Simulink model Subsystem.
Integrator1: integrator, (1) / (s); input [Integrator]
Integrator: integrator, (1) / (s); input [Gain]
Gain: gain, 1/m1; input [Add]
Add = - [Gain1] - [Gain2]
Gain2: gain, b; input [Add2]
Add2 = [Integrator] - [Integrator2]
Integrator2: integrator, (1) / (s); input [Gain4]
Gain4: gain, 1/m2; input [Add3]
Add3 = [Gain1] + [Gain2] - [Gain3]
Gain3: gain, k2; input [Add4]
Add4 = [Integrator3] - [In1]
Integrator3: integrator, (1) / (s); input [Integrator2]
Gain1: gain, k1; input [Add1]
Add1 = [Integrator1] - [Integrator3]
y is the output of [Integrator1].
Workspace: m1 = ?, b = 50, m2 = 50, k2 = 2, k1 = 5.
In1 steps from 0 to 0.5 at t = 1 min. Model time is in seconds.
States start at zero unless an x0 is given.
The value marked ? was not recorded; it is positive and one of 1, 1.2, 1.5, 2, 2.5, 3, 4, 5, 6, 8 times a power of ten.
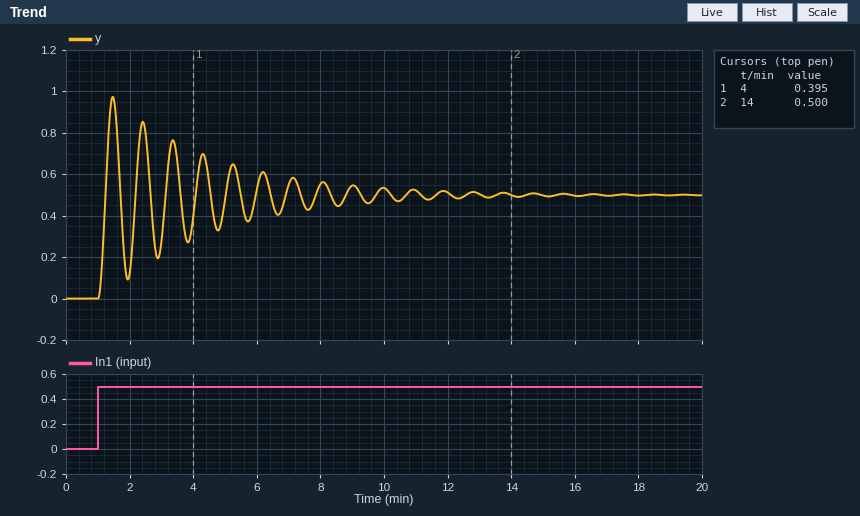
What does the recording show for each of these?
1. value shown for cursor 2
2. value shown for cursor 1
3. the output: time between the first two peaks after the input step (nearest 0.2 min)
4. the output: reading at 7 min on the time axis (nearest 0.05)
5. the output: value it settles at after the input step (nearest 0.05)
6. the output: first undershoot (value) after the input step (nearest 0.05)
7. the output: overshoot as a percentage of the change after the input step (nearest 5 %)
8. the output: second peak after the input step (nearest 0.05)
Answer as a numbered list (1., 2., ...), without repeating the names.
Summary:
1. 0.500
2. 0.395
3. 1.0 min
4. 0.55
5. 0.50
6. 0.10
7. 95 %
8. 0.85
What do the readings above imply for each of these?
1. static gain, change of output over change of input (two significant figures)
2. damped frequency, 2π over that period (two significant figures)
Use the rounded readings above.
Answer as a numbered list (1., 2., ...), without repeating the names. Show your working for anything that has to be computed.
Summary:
1. (0.5 - 0) / (0.5 - 0) = 1.0
2. 2π / 1 = 6.3 rad/min
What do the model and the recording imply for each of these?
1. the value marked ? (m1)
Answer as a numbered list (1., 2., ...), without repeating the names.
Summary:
1. 100
